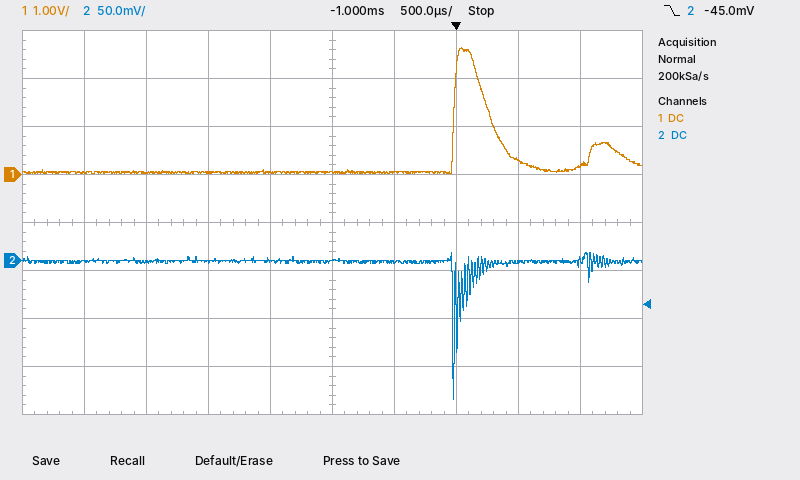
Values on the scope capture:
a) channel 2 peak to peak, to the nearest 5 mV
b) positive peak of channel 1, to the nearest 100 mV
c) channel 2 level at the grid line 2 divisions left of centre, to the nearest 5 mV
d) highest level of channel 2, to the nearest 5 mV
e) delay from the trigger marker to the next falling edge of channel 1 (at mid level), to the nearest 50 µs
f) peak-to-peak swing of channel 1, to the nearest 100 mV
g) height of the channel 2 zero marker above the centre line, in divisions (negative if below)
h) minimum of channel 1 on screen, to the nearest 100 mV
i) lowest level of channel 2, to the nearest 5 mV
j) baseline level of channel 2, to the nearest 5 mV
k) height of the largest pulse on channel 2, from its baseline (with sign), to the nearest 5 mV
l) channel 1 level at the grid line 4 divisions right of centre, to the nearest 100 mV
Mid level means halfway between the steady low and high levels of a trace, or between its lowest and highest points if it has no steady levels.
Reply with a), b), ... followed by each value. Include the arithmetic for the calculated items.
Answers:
a) 10 mV − (-145 mV) = 155 mV
b) 2.6 V
c) 0 mV
d) 10 mV
e) 250 µs
f) 2.6 V − (0.0 V) = 2.6 V
g) -0.8 div
h) 0.0 V
i) -145 mV
j) 0 mV
k) -145 mV − (0 mV) = -145 mV
l) 200 mV
